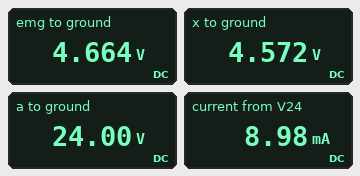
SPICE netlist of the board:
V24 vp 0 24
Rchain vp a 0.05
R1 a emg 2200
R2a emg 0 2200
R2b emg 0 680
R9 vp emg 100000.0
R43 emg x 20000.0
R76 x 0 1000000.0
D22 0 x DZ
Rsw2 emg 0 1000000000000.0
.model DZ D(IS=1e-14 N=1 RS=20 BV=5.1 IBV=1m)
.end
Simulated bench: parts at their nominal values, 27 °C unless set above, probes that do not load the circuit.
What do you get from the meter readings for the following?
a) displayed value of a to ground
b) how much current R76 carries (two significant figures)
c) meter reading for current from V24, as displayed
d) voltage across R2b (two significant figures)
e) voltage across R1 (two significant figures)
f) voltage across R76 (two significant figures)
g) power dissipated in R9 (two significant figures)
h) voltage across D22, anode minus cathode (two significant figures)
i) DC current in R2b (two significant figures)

24.00 V
4.6 µA
8.98 mA
4.7 V
19 V
4.6 V
3.7 mW
-4.6 V
6.9 mA
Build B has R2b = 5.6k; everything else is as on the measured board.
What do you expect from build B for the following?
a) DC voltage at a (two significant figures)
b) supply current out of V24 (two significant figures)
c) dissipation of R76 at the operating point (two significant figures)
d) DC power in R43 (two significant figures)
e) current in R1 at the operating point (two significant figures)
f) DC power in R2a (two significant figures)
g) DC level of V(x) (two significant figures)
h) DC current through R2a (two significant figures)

24 V
6.5 mA
26 µW
1.2 mW
6.4 mA
45 mW
5.1 V
4.5 mA
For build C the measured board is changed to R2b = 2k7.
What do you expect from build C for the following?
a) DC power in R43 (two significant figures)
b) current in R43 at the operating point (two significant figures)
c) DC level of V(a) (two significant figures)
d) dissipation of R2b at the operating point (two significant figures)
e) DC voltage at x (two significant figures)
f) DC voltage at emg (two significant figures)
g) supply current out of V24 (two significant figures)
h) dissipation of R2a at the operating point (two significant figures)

600 µW
170 µA
24 V
27 mW
5.1 V
8.5 V
7.2 mA
33 mW
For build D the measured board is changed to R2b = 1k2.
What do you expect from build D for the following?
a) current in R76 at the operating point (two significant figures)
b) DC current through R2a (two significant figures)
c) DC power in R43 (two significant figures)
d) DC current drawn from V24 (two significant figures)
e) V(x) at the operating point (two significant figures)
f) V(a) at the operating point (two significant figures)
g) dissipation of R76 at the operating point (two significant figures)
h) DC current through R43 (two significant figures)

5.0 µA
2.9 mA
84 µW
8.2 mA
5.0 V
24 V
25 µW
65 µA
